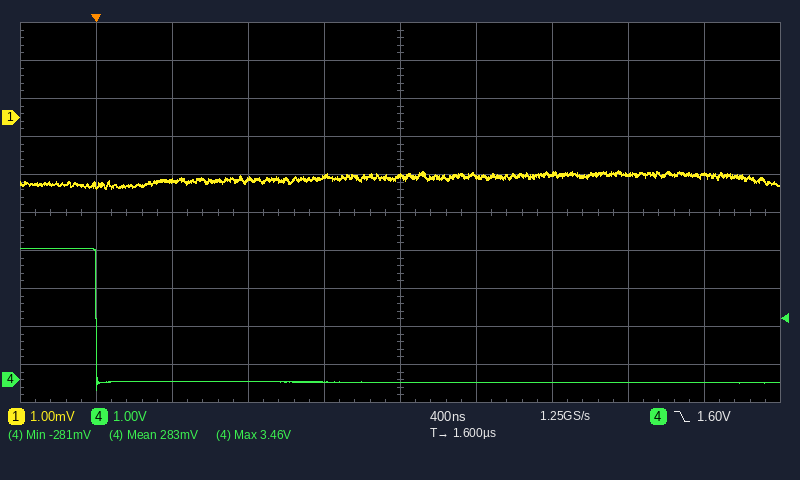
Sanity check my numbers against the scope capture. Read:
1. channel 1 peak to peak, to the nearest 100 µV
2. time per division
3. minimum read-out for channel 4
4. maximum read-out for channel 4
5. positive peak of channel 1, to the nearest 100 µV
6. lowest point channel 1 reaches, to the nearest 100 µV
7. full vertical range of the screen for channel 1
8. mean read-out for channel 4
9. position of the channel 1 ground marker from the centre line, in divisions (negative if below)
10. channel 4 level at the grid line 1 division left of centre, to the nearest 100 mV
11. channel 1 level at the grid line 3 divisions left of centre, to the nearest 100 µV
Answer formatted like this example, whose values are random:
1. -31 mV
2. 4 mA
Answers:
1. 500 µV
2. 400 ns
3. -281 mV
4. 3.46 V
5. -1.4 mV
6. -1.9 mV
7. 10 mV
8. 283 mV
9. +2.5 div
10. -100 mV
11. -1.7 mV
